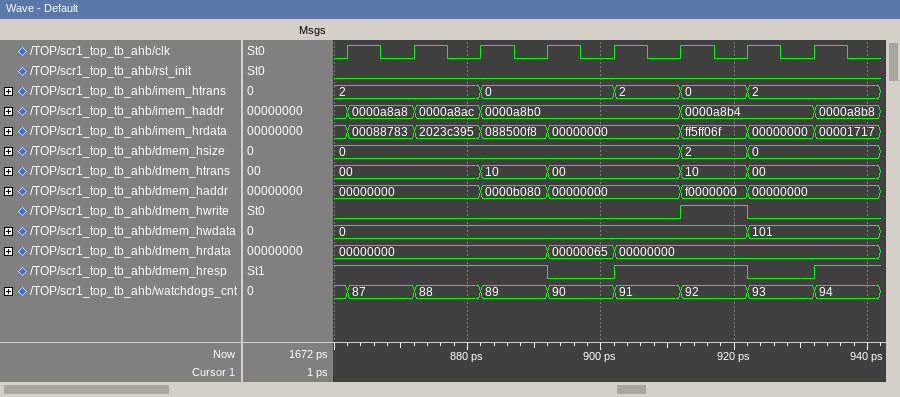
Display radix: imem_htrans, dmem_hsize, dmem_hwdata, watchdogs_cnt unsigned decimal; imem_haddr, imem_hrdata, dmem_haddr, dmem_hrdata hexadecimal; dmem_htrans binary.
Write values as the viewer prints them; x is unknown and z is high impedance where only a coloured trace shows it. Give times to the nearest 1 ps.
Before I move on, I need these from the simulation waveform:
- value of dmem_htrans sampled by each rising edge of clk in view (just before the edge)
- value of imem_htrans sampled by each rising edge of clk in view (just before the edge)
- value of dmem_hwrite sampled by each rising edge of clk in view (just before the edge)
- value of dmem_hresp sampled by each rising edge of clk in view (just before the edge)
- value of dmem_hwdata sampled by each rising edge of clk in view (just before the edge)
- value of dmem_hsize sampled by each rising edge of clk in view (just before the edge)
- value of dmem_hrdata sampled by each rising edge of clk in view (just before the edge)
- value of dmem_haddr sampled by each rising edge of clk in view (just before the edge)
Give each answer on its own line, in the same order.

00, 00, 00, 10, 00, 00, 10, 00
2, 2, 2, 0, 0, 2, 0, 2
0 0 0 0 0 0 1 0
1 1 1 1 0 1 1 0
0, 0, 0, 0, 0, 0, 0, 101
0, 0, 0, 0, 0, 0, 2, 0
00000000, 00000000, 00000000, 00000000, 00000065, 00000000, 00000000, 00000000
00000000, 00000000, 00000000, 0000b080, 00000000, 00000000, f0000000, 00000000
